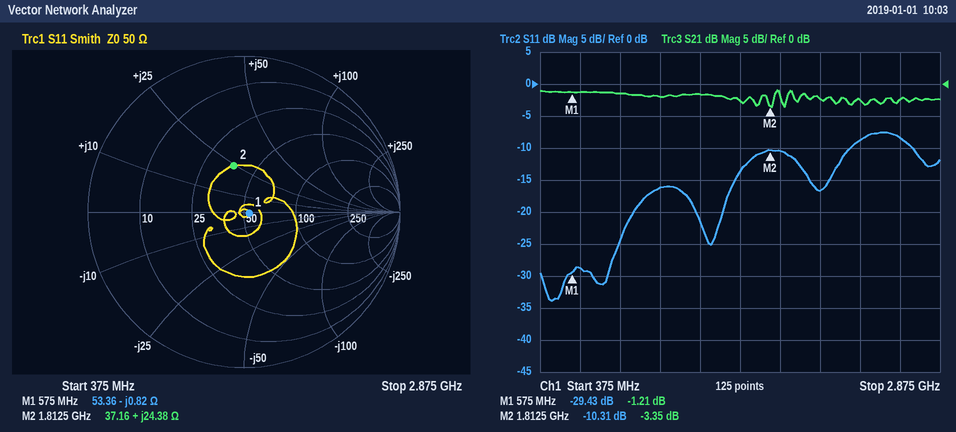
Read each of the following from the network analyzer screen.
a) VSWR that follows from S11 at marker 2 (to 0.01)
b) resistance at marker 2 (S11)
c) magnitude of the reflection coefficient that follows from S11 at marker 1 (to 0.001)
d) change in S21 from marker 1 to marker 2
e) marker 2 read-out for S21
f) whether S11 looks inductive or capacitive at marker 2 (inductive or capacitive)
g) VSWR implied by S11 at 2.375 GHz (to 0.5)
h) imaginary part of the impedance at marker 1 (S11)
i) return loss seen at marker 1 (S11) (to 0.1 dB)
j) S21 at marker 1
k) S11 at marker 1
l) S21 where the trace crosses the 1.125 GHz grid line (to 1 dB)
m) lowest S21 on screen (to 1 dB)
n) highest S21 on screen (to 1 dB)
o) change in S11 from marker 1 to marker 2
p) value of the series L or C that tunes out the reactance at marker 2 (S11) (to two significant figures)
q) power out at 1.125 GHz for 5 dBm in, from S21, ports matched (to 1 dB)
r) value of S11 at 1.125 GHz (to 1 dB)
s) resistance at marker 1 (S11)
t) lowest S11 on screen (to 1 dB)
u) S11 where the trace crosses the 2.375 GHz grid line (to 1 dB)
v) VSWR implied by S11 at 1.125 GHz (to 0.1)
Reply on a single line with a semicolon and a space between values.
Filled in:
1.88; 37.16 Ω; 0.034; -2.14 dB; -3.35 dB; inductive; 2.0; -0.82 Ω; 29.5 dB; -1.21 dB; -29.43 dB; -2 dB; -4 dB; -1 dB; 19.12 dB; 3.6 pF; 3 dBm; -16 dB; 53.36 Ω; -34 dB; -9 dB; 1.4
